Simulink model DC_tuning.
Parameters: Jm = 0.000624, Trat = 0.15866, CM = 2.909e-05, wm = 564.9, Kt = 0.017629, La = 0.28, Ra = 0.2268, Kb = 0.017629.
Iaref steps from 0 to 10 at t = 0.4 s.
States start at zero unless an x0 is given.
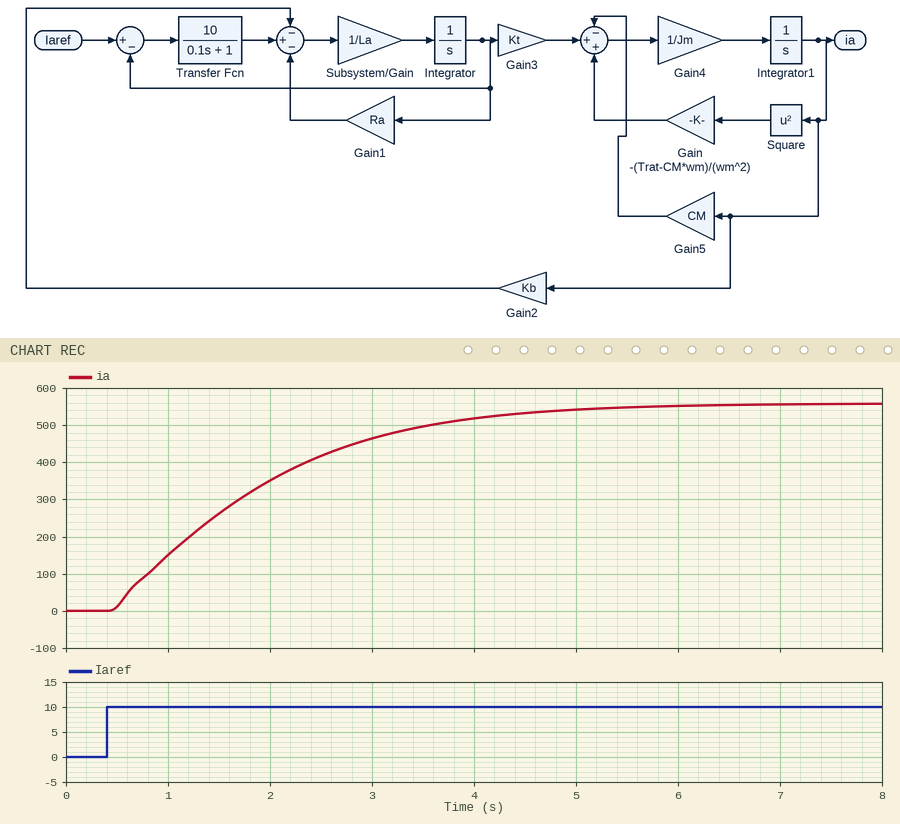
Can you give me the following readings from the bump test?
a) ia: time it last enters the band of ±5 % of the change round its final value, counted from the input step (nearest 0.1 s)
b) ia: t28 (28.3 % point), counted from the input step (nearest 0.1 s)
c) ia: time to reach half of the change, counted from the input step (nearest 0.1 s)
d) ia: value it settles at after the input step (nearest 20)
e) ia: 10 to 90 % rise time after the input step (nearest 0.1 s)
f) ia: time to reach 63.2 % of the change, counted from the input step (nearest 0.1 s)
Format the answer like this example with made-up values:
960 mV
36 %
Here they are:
4.0 s
0.6 s
1.2 s
560
3.0 s
1.6 s
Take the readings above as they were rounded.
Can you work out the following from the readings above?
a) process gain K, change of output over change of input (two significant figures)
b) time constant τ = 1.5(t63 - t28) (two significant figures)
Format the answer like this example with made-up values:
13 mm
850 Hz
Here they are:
56
1.5 s
